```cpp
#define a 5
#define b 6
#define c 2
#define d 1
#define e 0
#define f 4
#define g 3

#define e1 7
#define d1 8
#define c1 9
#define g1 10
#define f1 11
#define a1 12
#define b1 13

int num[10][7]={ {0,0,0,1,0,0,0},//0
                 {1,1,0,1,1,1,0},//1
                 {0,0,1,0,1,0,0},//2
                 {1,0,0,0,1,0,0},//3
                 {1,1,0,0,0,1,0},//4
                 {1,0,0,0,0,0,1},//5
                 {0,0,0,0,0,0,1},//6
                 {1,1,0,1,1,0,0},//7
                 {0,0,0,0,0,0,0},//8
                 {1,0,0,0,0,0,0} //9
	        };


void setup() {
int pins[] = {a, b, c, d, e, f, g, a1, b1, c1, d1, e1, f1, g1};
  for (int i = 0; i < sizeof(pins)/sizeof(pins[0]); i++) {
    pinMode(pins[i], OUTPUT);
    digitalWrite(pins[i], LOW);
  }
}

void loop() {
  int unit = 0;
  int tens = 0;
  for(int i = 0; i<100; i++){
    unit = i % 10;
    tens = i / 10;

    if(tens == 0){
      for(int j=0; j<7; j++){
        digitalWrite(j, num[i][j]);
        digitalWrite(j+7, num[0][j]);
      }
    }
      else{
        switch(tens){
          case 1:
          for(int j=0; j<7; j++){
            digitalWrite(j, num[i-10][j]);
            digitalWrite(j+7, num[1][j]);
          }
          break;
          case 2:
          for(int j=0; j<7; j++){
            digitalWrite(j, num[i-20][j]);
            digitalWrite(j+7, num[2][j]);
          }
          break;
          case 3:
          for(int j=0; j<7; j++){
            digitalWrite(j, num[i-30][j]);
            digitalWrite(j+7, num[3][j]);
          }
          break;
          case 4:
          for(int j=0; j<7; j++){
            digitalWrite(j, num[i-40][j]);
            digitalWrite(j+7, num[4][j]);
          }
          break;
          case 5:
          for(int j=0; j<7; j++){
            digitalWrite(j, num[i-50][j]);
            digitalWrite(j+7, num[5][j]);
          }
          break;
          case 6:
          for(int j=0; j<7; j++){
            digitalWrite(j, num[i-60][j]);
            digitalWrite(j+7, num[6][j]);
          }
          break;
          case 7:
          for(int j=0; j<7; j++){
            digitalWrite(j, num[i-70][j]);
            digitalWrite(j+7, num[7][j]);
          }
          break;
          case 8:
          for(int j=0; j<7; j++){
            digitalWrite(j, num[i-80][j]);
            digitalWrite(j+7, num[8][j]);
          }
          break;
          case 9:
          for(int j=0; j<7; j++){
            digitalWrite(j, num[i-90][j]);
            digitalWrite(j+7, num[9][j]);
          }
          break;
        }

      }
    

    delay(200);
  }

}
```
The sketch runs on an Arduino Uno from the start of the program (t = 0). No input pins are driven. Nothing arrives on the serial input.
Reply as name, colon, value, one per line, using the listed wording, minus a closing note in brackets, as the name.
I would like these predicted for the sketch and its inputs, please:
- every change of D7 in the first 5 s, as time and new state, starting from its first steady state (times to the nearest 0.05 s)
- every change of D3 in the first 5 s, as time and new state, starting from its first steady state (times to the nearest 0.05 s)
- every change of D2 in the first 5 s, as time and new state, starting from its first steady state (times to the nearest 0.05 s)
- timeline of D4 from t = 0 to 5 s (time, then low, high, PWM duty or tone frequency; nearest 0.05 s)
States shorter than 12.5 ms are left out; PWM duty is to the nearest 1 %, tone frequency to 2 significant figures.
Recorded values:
every change of D7 in the first 5 s, as time and new state, starting from its first steady state: 0 s low; 2 s high; 4 s low
every change of D3 in the first 5 s, as time and new state, starting from its first steady state: 0 s high; 0.4 s low; 1.4 s high; 1.6 s low; 2 s high; 2.4 s low; 3.4 s high; 3.6 s low; 4 s high; 4.4 s low
every change of D2 in the first 5 s, as time and new state, starting from its first steady state: 0 s low; 0.4 s high; 0.6 s low; 2.4 s high; 2.6 s low; 4.4 s high; 4.6 s low
timeline of D4 from t = 0 to 5 s: 0 s low; 0.2 s high; 0.8 s low; 1.4 s high; 1.6 s low; 2.2 s high; 2.8 s low; 3.4 s high; 3.6 s low; 4.2 s high; 4.8 s low
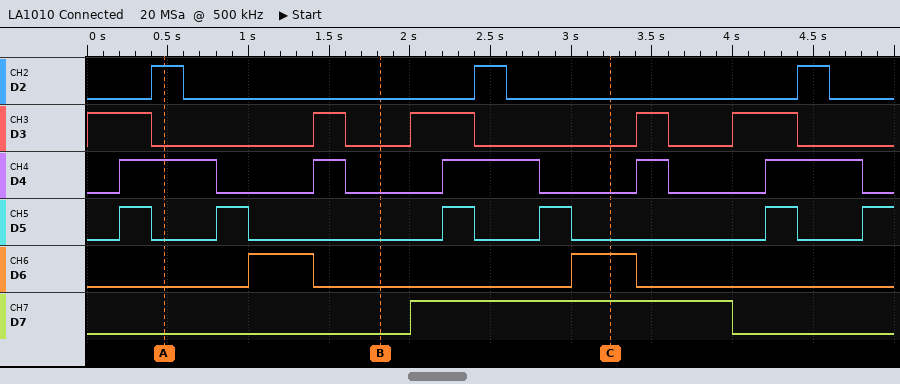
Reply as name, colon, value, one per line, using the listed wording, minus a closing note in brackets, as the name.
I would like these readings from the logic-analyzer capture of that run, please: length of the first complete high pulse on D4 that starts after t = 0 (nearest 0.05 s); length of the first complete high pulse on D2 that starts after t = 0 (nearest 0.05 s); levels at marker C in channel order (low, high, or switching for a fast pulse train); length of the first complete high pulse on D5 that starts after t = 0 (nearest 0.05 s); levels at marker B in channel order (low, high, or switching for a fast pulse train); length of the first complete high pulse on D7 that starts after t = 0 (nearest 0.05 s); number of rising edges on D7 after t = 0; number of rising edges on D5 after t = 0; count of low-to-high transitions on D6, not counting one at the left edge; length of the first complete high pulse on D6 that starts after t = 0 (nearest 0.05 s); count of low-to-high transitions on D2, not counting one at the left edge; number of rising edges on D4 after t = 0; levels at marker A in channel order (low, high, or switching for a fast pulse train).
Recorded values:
length of the first complete high pulse on D4 that starts after t = 0: 0.60 s
length of the first complete high pulse on D2 that starts after t = 0: 0.20 s
levels at marker C in channel order: D2 low, D3 low, D4 low, D5 low, D6 high, D7 high
length of the first complete high pulse on D5 that starts after t = 0: 0.20 s
levels at marker B in channel order: D2 low, D3 low, D4 low, D5 low, D6 low, D7 low
length of the first complete high pulse on D7 that starts after t = 0: 2.00 s
number of rising edges on D7 after t = 0: 1
number of rising edges on D5 after t = 0: 6
count of low-to-high transitions on D6, not counting one at the left edge: 2
length of the first complete high pulse on D6 that starts after t = 0: 0.40 s
count of low-to-high transitions on D2, not counting one at the left edge: 3
number of rising edges on D4 after t = 0: 5
levels at marker A in channel order: D2 high, D3 low, D4 high, D5 low, D6 low, D7 low
